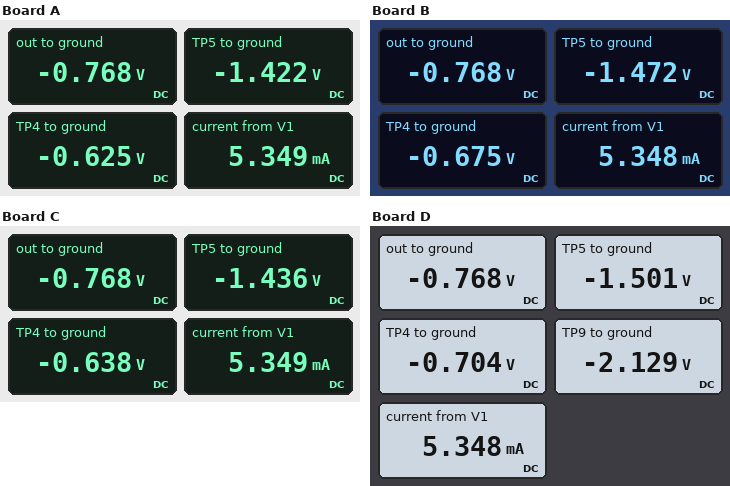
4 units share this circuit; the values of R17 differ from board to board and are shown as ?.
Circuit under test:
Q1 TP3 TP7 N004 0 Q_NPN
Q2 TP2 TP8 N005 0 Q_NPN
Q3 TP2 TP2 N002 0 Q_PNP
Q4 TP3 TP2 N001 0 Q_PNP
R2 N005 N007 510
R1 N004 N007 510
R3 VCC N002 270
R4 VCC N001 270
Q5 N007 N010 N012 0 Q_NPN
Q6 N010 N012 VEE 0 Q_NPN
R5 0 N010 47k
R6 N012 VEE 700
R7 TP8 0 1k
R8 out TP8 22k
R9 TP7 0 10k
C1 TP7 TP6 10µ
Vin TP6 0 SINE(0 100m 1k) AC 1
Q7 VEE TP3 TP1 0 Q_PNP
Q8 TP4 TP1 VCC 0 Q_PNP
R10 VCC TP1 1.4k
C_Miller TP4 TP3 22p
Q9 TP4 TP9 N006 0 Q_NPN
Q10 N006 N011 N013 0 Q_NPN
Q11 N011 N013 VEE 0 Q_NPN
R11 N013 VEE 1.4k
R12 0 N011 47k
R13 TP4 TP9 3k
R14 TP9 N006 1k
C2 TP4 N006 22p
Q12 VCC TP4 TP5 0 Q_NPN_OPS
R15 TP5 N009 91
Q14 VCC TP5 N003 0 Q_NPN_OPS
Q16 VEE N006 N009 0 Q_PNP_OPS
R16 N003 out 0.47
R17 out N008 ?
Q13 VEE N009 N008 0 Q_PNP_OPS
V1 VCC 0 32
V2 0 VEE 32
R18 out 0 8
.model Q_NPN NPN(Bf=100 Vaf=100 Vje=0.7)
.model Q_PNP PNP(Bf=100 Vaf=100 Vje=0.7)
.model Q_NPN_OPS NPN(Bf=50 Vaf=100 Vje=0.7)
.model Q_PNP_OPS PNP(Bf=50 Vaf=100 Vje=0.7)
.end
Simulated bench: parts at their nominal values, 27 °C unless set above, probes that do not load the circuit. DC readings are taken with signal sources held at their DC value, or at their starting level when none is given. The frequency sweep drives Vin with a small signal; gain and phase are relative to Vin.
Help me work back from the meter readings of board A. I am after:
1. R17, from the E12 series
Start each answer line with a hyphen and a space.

- 0.68 Ω
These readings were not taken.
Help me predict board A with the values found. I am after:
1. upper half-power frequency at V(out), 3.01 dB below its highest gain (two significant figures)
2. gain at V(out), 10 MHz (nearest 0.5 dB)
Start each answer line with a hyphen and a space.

- 460 kHz
- 1.0 dB
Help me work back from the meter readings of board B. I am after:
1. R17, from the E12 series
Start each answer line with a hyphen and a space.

- 1.2 Ω
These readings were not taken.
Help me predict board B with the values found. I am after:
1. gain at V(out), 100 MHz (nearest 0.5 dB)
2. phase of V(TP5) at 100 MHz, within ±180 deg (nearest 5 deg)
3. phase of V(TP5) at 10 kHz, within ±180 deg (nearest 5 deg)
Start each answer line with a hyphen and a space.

- -17.5 dB
- -125 deg
- 0 deg
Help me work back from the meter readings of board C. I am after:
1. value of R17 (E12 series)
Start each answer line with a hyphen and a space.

- 0.82 Ω
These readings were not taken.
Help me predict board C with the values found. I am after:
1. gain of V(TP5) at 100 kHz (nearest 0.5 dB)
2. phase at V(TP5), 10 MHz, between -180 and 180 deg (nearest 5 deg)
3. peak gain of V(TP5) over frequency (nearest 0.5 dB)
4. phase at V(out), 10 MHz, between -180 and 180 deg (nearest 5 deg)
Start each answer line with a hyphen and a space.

- 28.5 dB
- -90 deg
- 29.0 dB
- -90 deg
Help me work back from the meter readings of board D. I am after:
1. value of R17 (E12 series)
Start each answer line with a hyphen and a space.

- 1.5 Ω
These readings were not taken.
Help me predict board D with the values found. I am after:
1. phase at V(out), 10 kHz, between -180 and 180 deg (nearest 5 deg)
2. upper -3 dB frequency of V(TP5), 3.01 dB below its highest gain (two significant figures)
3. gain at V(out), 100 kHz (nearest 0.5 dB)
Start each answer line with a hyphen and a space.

- 0 deg
- 420 kHz
- 27.0 dB
